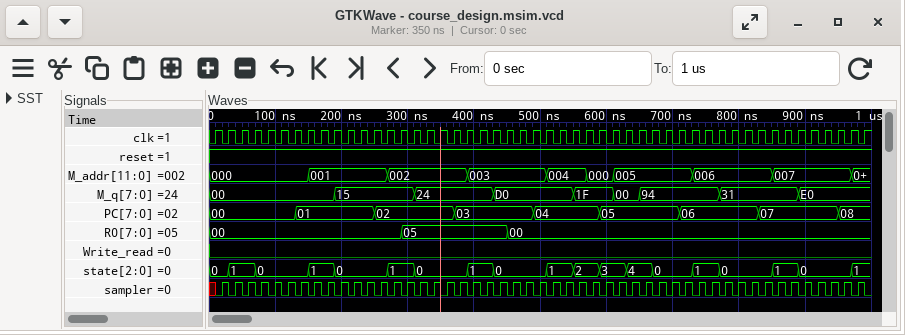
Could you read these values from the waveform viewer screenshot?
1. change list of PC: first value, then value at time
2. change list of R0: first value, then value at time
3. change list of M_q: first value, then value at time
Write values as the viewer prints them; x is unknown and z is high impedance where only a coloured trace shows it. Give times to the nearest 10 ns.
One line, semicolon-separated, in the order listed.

00, 01 at 130 ns, 02 at 250 ns, 03 at 370 ns, 04 at 490 ns, 05 at 590 ns, 06 at 710 ns, 07 at 830 ns, 08 at 950 ns; 00, 05 at 290 ns, 00 at 450 ns; 00, 15 at 190 ns, 24 at 310 ns, D0 at 430 ns, 1F at 550 ns, 00 at 610 ns, 94 at 650 ns, 31 at 770 ns, E0 at 890 ns
